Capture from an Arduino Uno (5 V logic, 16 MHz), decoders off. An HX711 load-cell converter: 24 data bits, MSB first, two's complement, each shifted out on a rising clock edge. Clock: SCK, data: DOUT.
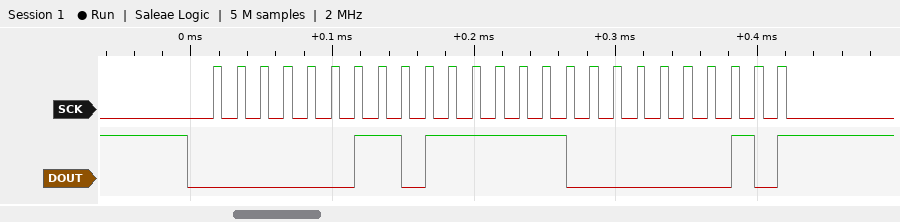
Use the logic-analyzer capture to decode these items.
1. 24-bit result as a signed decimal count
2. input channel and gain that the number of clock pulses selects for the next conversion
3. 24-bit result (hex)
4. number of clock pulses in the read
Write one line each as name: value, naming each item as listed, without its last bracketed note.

24-bit result as a signed decimal count: 228866
input channel and gain that the number of clock pulses selects for the next conversion: channel A, gain 128
24-bit result: 0x037E02
number of clock pulses in the read: 25
